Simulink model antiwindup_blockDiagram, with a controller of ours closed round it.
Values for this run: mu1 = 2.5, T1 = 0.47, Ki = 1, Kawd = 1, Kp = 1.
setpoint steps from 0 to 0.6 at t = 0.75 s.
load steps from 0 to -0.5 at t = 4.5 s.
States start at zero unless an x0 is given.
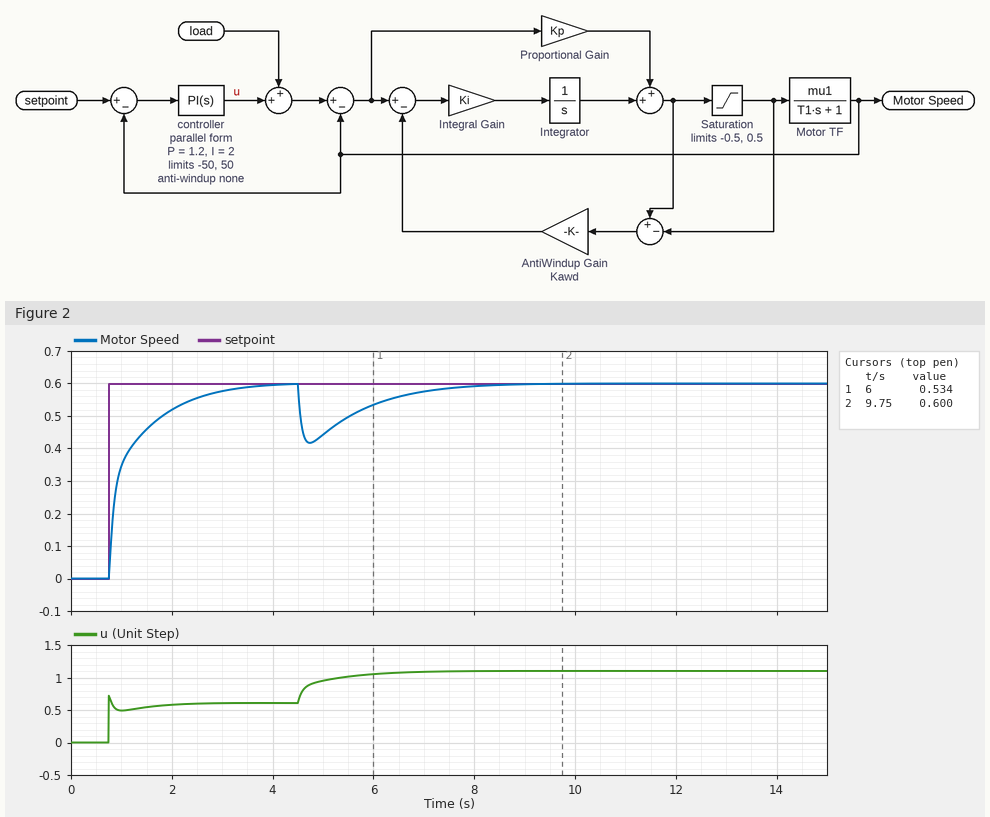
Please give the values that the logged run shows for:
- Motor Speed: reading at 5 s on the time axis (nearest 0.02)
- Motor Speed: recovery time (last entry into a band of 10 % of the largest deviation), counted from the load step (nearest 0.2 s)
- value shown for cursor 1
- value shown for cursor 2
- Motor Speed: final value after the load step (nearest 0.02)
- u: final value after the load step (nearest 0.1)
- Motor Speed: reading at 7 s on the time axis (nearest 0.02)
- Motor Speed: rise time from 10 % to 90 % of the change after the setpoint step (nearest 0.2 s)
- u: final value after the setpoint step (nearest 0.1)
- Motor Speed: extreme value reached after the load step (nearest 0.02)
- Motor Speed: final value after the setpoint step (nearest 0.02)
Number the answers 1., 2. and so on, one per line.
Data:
1. 0.44
2. 2.8 s
3. 0.534
4. 0.600
5. 0.60
6. 1.1
7. 0.58
8. 1.4 s
9. 0.6
10. 0.42
11. 0.60
